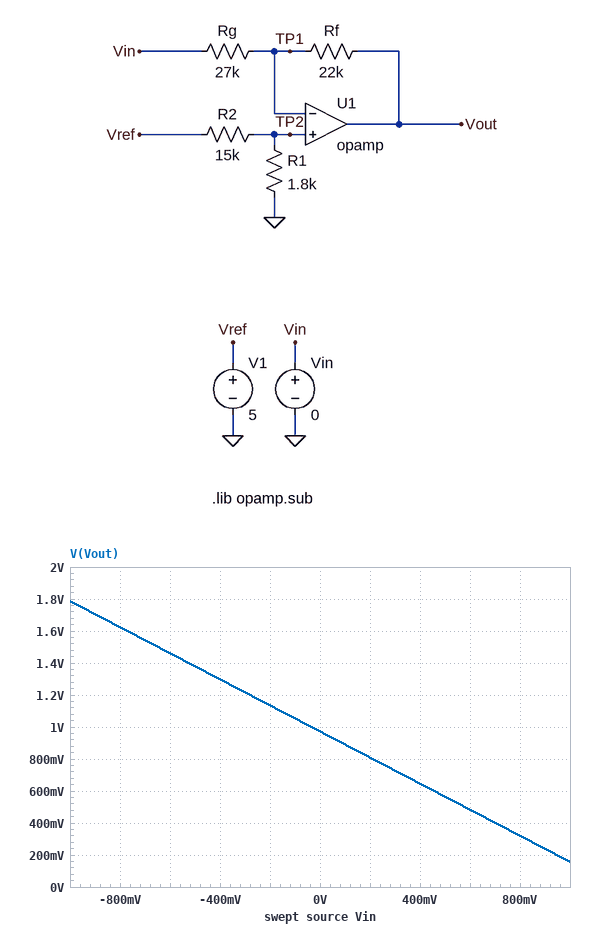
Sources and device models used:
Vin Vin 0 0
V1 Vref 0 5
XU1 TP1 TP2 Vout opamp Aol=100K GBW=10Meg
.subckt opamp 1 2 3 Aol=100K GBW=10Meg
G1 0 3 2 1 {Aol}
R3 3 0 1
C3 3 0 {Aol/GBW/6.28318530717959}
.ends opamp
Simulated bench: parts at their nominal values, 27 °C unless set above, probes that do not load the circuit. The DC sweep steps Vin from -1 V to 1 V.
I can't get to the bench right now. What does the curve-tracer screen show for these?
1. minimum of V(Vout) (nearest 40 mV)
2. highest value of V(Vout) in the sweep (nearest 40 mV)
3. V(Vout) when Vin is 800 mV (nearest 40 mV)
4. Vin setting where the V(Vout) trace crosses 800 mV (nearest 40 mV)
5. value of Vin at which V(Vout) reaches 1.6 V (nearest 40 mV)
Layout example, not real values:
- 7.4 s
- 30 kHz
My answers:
- 160 mV
- 1.80 V
- 320 mV
- 200 mV
- -760 mV
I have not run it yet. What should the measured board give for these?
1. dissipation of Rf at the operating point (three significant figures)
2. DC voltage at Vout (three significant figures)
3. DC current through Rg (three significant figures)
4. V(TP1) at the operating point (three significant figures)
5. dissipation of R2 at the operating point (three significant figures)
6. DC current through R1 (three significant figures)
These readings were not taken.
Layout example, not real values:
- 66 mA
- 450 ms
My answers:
- 8.66 µW
- 972 mV
- 19.8 µA
- 536 mV
- 1.33 mW
- 298 µA
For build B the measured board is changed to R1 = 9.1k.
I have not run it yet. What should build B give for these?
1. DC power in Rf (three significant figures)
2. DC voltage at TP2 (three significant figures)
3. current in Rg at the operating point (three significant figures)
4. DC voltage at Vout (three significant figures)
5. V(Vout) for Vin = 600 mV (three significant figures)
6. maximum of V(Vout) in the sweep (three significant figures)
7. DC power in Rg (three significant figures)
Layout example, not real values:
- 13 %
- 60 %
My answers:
- 108 µW
- 1.89 V
- 69.9 µA
- 3.43 V
- 2.94 V
- 4.24 V
- 132 µW
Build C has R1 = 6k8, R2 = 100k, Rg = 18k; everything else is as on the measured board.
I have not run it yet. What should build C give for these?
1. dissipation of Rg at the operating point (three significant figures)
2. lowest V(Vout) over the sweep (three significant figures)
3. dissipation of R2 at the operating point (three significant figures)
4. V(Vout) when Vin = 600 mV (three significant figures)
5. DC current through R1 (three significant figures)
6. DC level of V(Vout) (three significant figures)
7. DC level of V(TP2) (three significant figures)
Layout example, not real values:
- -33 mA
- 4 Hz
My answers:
- 5.63 µW
- -515 mV
- 219 µW
- -25.9 mV
- 46.8 µA
- 707 mV
- 318 mV
